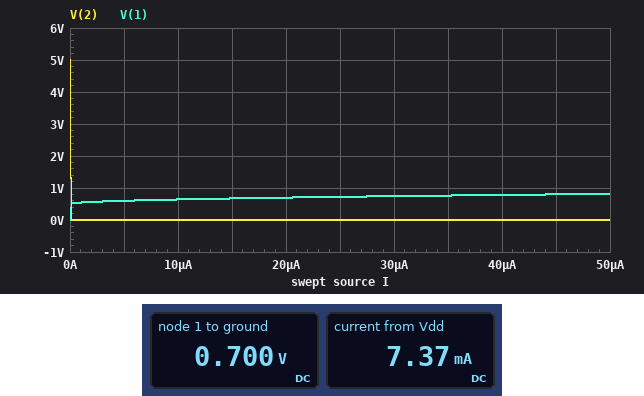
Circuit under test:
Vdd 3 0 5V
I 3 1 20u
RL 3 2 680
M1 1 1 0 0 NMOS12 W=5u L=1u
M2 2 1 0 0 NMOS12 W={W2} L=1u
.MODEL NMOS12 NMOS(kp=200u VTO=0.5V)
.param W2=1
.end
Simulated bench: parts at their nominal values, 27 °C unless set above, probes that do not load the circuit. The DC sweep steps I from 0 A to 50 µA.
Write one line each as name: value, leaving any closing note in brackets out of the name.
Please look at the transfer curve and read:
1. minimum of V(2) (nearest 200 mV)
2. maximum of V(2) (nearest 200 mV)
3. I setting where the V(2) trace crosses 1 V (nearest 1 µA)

minimum of V(2): 0 V
maximum of V(2): 5.0 V
I setting where the V(2) trace crosses 1 V: 0 A
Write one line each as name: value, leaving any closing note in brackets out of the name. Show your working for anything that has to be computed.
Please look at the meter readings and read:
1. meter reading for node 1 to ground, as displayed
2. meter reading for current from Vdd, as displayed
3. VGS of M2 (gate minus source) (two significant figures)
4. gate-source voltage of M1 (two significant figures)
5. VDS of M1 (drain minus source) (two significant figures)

meter reading for node 1 to ground, as displayed: 0.700 V
meter reading for current from Vdd, as displayed: 7.37 mA
VGS of M2 (gate minus source): 700 mV = 700 mV
gate-source voltage of M1: 700 mV = 700 mV
VDS of M1 (drain minus source): 700 mV = 700 mV
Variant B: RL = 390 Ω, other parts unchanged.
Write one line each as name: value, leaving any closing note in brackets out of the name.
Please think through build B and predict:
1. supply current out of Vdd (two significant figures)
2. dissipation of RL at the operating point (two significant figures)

supply current out of Vdd: 13 mA
dissipation of RL at the operating point: 64 mW
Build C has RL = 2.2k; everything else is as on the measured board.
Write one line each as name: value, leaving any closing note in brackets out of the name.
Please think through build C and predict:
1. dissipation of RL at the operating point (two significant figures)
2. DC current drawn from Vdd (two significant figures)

dissipation of RL at the operating point: 11 mW
DC current drawn from Vdd: 2.3 mA
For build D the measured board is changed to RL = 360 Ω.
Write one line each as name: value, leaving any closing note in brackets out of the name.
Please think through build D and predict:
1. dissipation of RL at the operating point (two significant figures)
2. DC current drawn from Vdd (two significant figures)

dissipation of RL at the operating point: 69 mW
DC current drawn from Vdd: 14 mA
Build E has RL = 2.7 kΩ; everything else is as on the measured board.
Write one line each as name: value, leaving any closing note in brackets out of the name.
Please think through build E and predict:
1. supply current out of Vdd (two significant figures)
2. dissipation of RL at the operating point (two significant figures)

supply current out of Vdd: 1.9 mA
dissipation of RL at the operating point: 9.3 mW
